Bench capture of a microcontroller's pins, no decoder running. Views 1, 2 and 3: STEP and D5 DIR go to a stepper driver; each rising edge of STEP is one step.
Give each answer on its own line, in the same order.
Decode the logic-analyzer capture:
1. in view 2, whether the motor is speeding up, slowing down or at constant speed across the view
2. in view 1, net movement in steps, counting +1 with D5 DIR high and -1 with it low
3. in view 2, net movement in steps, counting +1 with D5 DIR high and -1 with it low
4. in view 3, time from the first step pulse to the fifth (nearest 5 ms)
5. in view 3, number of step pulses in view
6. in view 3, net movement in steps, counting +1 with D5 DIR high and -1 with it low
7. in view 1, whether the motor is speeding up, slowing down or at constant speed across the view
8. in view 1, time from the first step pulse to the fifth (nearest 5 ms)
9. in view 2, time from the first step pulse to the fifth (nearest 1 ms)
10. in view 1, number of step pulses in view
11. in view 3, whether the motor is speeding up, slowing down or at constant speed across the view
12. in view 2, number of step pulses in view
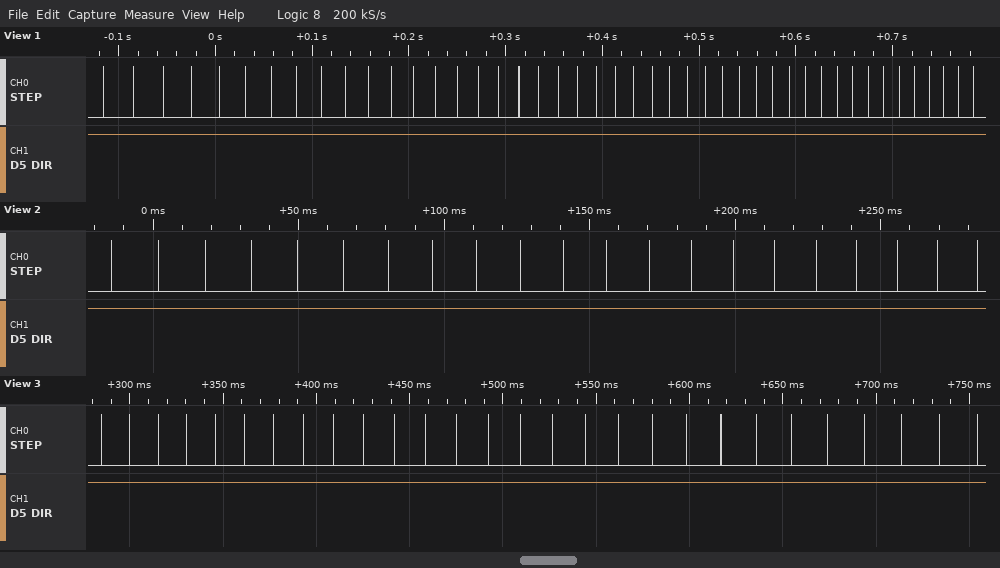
speeding up
+45
+21
60 ms
28
+28
speeding up
120 ms
64 ms
45
slowing down
21
